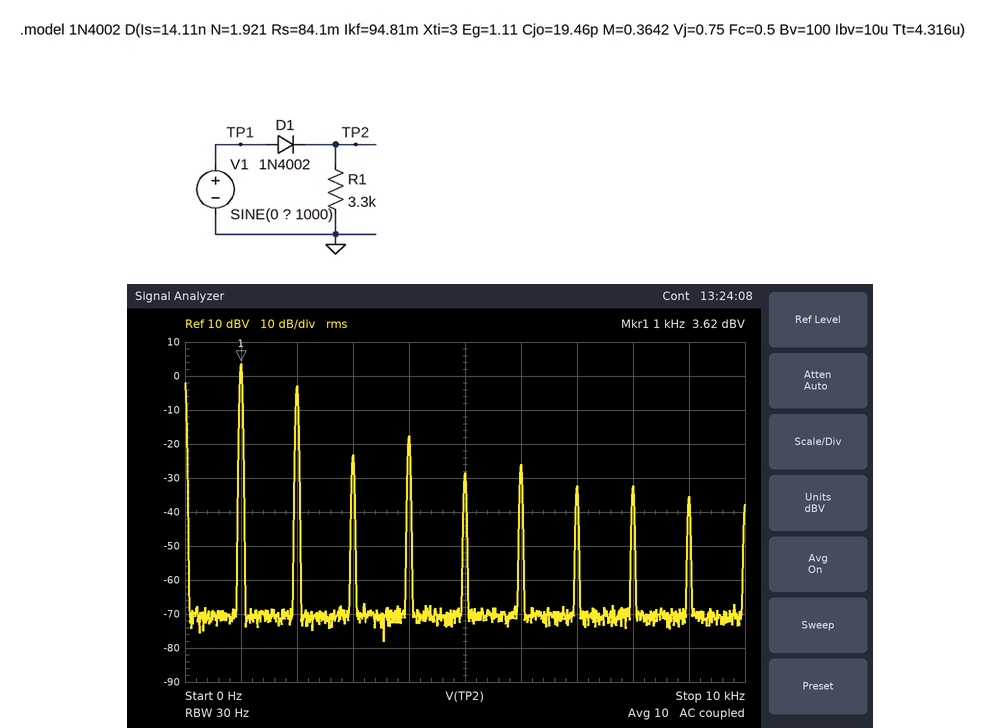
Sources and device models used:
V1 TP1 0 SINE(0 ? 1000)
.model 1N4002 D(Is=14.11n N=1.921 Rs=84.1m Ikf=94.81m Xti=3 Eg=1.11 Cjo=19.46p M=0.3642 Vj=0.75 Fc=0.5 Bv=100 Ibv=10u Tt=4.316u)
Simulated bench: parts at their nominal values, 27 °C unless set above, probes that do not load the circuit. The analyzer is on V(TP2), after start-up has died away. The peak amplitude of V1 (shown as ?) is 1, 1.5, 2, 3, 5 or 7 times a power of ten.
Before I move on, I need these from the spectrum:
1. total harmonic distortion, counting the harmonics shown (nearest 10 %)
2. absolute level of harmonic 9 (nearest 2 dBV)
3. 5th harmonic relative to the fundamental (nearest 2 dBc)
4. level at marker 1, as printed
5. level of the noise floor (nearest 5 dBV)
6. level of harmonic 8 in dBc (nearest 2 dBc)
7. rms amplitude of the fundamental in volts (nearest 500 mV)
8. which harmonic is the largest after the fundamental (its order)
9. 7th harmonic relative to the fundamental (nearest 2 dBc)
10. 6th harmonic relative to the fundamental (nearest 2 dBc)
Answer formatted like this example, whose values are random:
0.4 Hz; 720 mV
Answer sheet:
50 %; -36 dBV; -32 dBc; 3.62 dBV; -70 dBV; -36 dBc; 1.5 V; 2; -36 dBc; -30 dBc
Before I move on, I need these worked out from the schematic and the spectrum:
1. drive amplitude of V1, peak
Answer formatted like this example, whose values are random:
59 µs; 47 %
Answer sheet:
5 V
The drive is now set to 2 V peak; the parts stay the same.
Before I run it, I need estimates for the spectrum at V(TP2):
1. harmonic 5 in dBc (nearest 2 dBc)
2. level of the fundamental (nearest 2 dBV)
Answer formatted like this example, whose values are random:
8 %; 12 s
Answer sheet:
-26 dBc; -6 dBV
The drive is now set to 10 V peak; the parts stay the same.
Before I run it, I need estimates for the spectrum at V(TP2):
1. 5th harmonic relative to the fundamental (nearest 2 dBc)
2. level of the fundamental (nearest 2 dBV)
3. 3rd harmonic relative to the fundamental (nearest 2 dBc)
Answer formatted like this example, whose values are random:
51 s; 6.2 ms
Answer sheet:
-38 dBc; 10 dBV; -32 dBc
